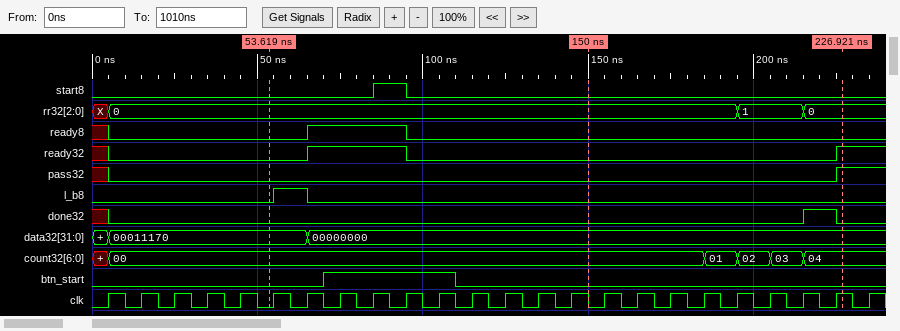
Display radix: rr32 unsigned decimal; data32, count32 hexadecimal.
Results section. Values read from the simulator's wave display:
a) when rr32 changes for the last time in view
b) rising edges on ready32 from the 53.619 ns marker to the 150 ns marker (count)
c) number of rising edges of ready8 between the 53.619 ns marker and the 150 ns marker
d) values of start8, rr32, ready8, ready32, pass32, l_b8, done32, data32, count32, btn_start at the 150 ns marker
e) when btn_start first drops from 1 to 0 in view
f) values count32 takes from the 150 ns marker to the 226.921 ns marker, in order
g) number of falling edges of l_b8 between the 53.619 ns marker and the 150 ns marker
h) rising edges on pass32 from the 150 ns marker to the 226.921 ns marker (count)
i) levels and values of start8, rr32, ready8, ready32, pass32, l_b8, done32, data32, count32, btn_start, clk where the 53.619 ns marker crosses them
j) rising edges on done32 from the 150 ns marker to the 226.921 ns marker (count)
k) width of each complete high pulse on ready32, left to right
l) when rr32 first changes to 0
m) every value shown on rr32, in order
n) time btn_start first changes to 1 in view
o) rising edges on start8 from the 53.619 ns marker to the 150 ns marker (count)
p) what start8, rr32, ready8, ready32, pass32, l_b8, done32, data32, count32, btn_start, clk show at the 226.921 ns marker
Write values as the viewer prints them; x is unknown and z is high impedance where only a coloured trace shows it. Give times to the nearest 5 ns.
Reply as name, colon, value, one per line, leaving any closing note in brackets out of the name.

when rr32 changes for the last time in view: 215 ns
rising edges on ready32 from the 53.619 ns marker to the 150 ns marker: 1
number of rising edges of ready8 between the 53.619 ns marker and the 150 ns marker: 1
values of start8, rr32, ready8, ready32, pass32, l_b8, done32, data32, count32, btn_start at the 150 ns marker: start8=0, rr32=0, ready8=0, ready32=0, pass32=0, l_b8=0, done32=0, data32=00000000, count32=00, btn_start=0
when btn_start first drops from 1 to 0 in view: 110 ns
values count32 takes from the 150 ns marker to the 226.921 ns marker, in order: 00, 01, 02, 03, 04
number of falling edges of l_b8 between the 53.619 ns marker and the 150 ns marker: 1
rising edges on pass32 from the 150 ns marker to the 226.921 ns marker: 1
levels and values of start8, rr32, ready8, ready32, pass32, l_b8, done32, data32, count32, btn_start, clk where the 53.619 ns marker crosses them: start8=0, rr32=0, ready8=0, ready32=0, pass32=0, l_b8=0, done32=0, data32=00011170, count32=00, btn_start=0, clk=0
rising edges on done32 from the 150 ns marker to the 226.921 ns marker: 1
width of each complete high pulse on ready32, left to right: 30 ns
when rr32 first changes to 0: 5 ns
every value shown on rr32, in order: X, 0, 1, 0
time btn_start first changes to 1 in view: 70 ns
rising edges on start8 from the 53.619 ns marker to the 150 ns marker: 1
what start8, rr32, ready8, ready32, pass32, l_b8, done32, data32, count32, btn_start, clk show at the 226.921 ns marker: start8=0, rr32=0, ready8=0, ready32=1, pass32=1, l_b8=0, done32=0, data32=00000000, count32=04, btn_start=0, clk=1
